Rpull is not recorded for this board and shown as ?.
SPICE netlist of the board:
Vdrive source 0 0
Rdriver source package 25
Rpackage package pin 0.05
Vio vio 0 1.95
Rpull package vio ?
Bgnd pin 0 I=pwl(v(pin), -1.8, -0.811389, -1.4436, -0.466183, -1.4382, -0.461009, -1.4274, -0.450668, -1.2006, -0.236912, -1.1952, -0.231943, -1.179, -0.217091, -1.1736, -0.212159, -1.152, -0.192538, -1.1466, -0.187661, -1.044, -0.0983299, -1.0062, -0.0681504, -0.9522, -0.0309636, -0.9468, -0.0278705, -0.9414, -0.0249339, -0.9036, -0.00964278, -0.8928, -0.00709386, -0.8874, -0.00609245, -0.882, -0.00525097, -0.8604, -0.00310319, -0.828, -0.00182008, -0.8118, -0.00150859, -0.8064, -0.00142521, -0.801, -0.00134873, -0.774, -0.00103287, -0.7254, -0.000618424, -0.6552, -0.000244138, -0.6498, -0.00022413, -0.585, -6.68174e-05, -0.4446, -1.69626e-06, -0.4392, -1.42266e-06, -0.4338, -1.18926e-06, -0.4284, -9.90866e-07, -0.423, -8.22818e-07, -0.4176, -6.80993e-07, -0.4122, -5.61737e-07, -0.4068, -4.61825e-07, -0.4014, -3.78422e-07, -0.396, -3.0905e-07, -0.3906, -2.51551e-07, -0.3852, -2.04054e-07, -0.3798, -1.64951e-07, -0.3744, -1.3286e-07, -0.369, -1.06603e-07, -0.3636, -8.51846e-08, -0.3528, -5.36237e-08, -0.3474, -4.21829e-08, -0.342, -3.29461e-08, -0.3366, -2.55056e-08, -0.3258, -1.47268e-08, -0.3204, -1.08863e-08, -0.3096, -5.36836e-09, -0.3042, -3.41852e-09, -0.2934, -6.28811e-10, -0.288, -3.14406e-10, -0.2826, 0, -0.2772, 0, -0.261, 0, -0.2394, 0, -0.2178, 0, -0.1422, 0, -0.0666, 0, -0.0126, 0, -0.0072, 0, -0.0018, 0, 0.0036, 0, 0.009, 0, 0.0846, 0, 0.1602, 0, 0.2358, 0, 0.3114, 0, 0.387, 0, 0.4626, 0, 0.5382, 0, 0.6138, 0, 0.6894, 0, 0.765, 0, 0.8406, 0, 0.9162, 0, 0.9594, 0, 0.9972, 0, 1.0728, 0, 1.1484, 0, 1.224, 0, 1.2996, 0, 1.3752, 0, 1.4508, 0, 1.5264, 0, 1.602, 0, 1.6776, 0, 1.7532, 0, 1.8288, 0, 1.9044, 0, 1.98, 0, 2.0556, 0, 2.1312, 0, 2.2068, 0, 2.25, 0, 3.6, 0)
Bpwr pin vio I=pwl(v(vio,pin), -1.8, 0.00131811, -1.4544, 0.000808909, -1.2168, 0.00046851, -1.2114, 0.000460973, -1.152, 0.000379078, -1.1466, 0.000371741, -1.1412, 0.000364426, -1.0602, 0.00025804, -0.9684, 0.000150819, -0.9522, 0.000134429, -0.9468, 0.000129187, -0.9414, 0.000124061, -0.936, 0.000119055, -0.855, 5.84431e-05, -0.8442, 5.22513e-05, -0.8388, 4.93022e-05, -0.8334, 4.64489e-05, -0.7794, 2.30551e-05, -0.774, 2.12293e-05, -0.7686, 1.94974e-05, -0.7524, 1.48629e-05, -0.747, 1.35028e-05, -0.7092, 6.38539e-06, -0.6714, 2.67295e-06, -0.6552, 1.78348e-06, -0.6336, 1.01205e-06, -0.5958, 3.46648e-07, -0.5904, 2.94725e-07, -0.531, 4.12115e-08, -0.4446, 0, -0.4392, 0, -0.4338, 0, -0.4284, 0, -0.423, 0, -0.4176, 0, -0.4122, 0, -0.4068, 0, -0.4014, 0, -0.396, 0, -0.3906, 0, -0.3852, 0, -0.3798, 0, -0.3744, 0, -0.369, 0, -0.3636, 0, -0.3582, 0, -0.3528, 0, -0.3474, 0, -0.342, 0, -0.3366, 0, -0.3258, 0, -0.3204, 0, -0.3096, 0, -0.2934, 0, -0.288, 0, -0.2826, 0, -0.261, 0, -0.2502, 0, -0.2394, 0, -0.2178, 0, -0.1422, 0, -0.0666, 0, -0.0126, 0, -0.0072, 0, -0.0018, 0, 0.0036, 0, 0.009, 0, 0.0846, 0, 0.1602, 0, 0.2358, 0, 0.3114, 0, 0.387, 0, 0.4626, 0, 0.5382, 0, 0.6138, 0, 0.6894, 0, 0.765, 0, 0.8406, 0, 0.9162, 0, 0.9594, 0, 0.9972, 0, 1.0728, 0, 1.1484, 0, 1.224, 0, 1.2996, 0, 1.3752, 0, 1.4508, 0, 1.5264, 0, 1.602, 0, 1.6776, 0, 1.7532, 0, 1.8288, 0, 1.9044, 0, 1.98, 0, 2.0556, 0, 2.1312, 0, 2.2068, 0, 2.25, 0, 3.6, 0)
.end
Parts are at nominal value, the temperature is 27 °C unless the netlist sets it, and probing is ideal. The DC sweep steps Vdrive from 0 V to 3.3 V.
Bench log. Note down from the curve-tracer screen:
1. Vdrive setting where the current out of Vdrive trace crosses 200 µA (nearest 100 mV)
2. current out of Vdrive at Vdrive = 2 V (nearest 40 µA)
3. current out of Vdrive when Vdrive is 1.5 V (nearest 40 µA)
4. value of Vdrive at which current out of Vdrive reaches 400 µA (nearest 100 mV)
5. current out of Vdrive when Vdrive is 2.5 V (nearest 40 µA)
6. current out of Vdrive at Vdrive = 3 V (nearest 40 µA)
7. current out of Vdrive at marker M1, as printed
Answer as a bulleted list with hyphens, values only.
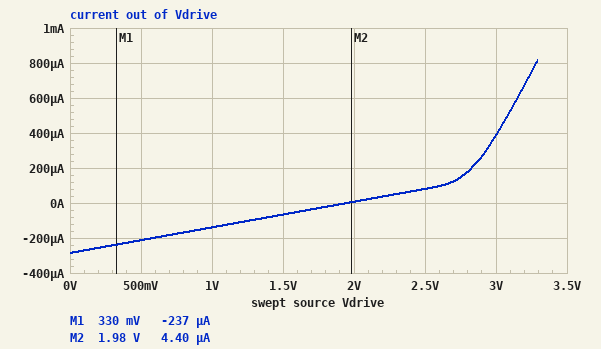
- 2.8 V
- 0 A
- -80 µA
- 3.0 V
- 80 µA
- 400 µA
- -237 µA
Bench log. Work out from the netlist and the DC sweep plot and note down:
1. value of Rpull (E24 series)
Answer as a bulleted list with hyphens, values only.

- 6.8 kΩ
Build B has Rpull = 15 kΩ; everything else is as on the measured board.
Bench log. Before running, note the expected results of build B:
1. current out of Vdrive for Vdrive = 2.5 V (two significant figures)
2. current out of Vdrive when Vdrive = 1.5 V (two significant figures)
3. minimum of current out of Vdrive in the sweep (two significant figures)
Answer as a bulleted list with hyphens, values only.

- 37 µA
- -30 µA
- -130 µA
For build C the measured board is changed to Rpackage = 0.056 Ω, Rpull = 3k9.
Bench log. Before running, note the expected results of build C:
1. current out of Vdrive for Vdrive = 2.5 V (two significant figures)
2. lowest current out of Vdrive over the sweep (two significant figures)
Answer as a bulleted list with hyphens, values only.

- 140 µA
- -500 µA
